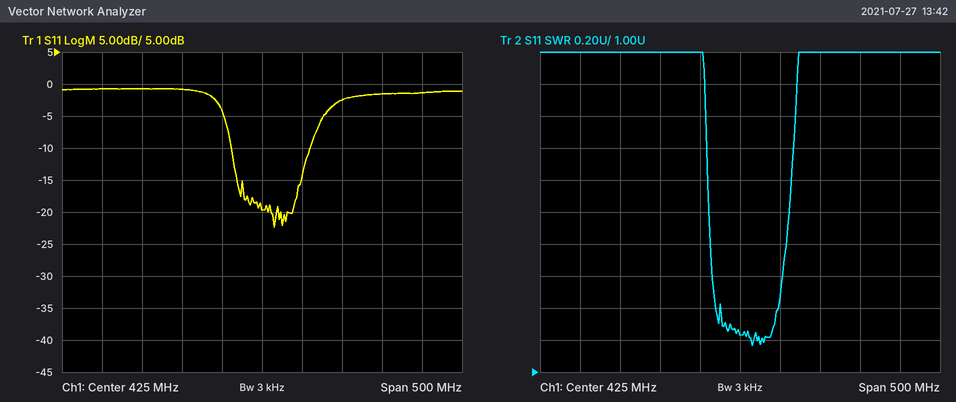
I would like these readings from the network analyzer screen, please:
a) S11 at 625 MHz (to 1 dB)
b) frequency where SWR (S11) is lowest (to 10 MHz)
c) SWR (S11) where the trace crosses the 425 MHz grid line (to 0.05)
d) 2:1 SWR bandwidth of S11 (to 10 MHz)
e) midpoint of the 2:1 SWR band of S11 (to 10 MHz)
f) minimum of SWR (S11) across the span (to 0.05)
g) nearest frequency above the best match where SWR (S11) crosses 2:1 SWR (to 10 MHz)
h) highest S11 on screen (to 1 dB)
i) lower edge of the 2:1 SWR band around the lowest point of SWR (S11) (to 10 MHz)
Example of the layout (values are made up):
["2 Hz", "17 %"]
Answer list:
["-1 dB", "440 MHz", "1.25", "100 MHz", "440 MHz", "1.15", "490 MHz", "-1 dB", "390 MHz"]
